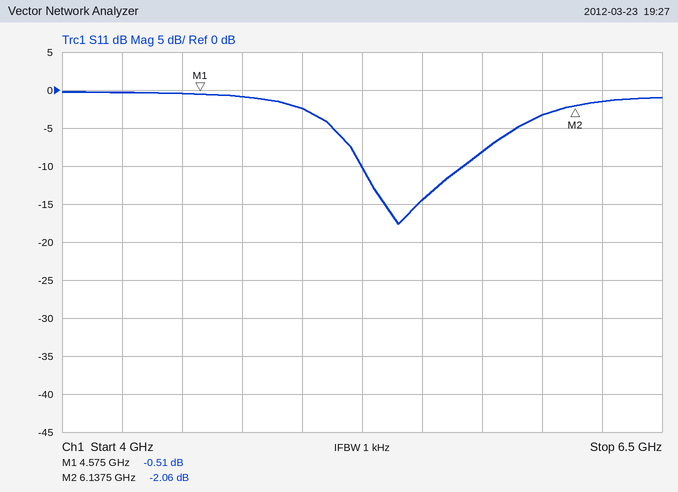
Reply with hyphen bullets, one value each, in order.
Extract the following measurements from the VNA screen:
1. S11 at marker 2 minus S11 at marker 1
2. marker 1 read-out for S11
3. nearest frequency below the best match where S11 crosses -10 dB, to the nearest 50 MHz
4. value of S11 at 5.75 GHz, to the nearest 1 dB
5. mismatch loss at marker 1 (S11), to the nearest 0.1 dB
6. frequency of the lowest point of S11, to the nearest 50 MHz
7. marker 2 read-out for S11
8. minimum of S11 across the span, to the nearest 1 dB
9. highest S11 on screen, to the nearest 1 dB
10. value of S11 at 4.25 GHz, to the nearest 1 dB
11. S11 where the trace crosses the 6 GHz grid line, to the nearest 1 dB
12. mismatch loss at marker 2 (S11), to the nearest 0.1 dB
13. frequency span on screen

- -1.55 dB
- -0.51 dB
- 5.25 GHz
- -8 dB
- 9.6 dB
- 5.40 GHz
- -2.06 dB
- -18 dB
- 0 dB
- 0 dB
- -3 dB
- 4.2 dB
- 2.5 GHz
